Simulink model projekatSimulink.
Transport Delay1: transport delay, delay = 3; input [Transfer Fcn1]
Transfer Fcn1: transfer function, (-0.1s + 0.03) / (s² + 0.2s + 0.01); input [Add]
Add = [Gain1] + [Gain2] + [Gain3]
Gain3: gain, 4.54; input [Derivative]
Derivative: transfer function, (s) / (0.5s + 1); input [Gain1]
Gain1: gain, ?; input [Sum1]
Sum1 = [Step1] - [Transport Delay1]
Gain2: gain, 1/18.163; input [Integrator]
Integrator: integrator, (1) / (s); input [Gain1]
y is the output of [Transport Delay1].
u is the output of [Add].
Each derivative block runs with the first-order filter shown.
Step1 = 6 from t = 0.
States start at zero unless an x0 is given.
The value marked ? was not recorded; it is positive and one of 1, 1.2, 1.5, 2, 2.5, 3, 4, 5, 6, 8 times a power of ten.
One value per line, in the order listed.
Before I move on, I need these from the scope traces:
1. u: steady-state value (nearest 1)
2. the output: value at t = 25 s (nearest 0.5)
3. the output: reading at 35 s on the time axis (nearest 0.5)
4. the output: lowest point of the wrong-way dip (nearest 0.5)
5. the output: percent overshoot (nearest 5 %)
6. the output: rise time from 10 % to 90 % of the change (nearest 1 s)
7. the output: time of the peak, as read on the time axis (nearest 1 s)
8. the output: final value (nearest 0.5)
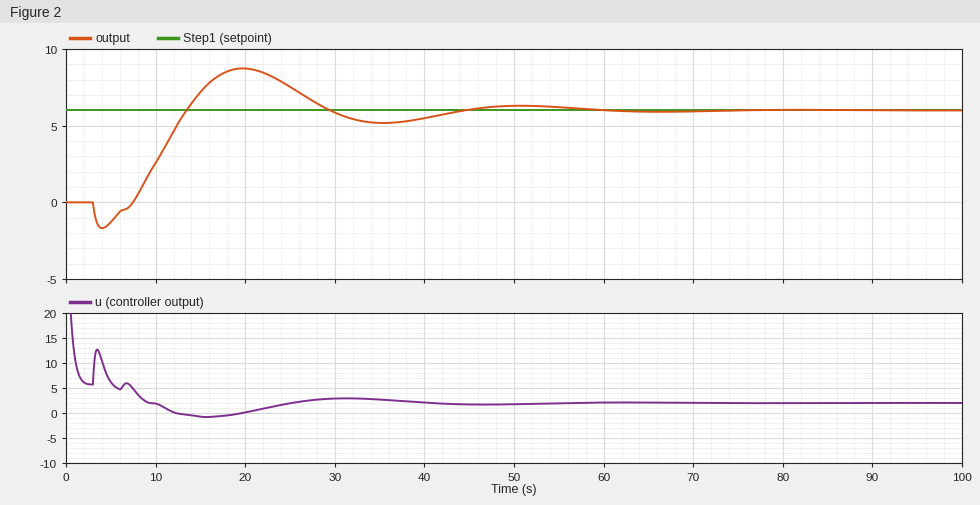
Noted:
2
7.5
5.0
-1.5
45 %
5 s
20 s
6.0
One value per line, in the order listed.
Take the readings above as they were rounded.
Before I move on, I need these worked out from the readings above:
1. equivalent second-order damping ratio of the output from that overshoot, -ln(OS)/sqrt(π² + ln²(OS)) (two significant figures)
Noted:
0.25
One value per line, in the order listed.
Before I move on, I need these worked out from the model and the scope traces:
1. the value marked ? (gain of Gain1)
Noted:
0.8
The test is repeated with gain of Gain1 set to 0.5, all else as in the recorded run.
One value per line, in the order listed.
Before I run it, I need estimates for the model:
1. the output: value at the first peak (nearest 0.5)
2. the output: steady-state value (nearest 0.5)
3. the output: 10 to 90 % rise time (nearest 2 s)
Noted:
6.5
6.0
10 s
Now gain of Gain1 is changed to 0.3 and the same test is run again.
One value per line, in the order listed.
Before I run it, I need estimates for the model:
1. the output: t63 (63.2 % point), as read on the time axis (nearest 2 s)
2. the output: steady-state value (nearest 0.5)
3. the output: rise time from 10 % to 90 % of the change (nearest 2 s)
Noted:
22 s
6.0
26 s
